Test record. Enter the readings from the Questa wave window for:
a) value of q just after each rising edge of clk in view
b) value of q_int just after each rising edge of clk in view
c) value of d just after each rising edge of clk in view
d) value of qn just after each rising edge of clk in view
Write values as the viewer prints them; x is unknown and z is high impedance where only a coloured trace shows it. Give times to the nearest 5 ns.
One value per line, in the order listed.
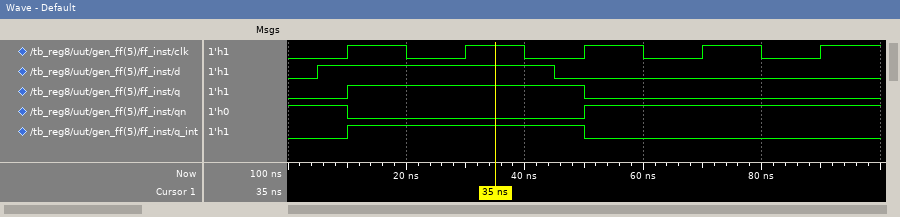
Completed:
1 1 0 0 0
1 1 0 0 0
1 1 0 0 0
0 0 1 1 1
